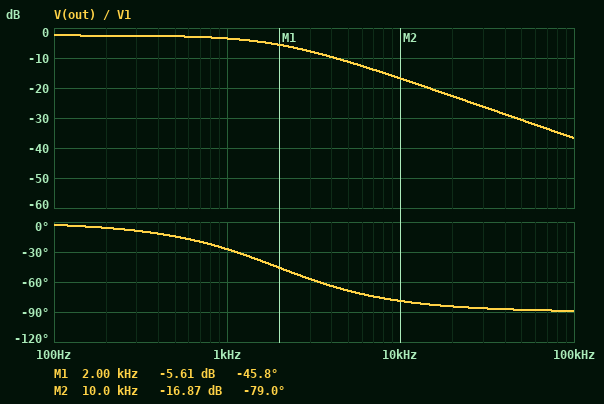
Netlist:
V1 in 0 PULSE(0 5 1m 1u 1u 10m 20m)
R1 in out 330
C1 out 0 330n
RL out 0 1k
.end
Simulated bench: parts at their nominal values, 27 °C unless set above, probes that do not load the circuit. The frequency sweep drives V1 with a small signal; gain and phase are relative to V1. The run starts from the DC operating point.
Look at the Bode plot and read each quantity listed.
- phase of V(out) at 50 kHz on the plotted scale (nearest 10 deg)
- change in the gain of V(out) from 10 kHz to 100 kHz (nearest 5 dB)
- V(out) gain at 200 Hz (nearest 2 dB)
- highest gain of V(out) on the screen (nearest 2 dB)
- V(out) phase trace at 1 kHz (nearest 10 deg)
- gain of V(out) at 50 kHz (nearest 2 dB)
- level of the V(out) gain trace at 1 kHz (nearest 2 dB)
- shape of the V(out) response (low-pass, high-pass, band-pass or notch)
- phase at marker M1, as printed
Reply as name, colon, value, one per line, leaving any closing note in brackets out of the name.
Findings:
phase of V(out) at 50 kHz on the plotted scale: -90 deg
change in the gain of V(out) from 10 kHz to 100 kHz: -20 dB
V(out) gain at 200 Hz: -2 dB
highest gain of V(out) on the screen: -2 dB
V(out) phase trace at 1 kHz: -30 deg
gain of V(out) at 50 kHz: -30 dB
level of the V(out) gain trace at 1 kHz: -4 dB
shape of the V(out) response: low-pass
phase at marker M1, as printed: -45.8 deg
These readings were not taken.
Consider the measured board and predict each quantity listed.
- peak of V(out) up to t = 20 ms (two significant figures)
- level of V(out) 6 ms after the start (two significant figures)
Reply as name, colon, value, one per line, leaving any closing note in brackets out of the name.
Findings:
peak of V(out) up to t = 20 ms: 3.8 V
level of V(out) 6 ms after the start: 3.8 V
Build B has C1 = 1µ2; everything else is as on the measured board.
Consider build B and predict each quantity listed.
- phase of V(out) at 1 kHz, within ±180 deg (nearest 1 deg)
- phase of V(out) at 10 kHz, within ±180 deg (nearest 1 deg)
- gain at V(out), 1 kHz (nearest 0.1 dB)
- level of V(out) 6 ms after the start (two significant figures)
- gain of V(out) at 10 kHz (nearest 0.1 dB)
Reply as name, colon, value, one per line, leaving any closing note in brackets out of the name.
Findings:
phase of V(out) at 1 kHz, within ±180 deg: -62 deg
phase of V(out) at 10 kHz, within ±180 deg: -87 deg
gain at V(out), 1 kHz: -9.0 dB
level of V(out) 6 ms after the start: 3.8 V
gain of V(out) at 10 kHz: -27.9 dB
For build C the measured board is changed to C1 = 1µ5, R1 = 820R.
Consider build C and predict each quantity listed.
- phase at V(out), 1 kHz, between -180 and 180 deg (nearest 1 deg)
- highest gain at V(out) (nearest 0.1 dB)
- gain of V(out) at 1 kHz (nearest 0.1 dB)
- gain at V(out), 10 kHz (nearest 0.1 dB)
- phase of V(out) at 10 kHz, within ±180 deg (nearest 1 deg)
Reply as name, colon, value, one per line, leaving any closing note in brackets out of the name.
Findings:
phase at V(out), 1 kHz, between -180 and 180 deg: -77 deg
highest gain at V(out): -5.2 dB
gain of V(out) at 1 kHz: -18.0 dB
gain at V(out), 10 kHz: -37.8 dB
phase of V(out) at 10 kHz, within ±180 deg: -89 deg
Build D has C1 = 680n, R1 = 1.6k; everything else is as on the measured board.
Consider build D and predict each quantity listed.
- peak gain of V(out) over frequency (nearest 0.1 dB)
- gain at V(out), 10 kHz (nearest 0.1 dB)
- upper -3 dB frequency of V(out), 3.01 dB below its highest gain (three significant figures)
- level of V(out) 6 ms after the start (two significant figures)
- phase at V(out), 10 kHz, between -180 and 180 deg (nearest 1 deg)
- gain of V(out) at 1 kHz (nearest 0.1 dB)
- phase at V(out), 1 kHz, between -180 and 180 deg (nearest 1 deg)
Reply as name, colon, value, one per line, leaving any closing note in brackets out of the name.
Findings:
peak gain of V(out) over frequency: -8.3 dB
gain at V(out), 10 kHz: -36.7 dB
upper -3 dB frequency of V(out), 3.01 dB below its highest gain: 380 Hz
level of V(out) 6 ms after the start: 1.9 V
phase at V(out), 10 kHz, between -180 and 180 deg: -88 deg
gain of V(out) at 1 kHz: -17.3 dB
phase at V(out), 1 kHz, between -180 and 180 deg: -69 deg
